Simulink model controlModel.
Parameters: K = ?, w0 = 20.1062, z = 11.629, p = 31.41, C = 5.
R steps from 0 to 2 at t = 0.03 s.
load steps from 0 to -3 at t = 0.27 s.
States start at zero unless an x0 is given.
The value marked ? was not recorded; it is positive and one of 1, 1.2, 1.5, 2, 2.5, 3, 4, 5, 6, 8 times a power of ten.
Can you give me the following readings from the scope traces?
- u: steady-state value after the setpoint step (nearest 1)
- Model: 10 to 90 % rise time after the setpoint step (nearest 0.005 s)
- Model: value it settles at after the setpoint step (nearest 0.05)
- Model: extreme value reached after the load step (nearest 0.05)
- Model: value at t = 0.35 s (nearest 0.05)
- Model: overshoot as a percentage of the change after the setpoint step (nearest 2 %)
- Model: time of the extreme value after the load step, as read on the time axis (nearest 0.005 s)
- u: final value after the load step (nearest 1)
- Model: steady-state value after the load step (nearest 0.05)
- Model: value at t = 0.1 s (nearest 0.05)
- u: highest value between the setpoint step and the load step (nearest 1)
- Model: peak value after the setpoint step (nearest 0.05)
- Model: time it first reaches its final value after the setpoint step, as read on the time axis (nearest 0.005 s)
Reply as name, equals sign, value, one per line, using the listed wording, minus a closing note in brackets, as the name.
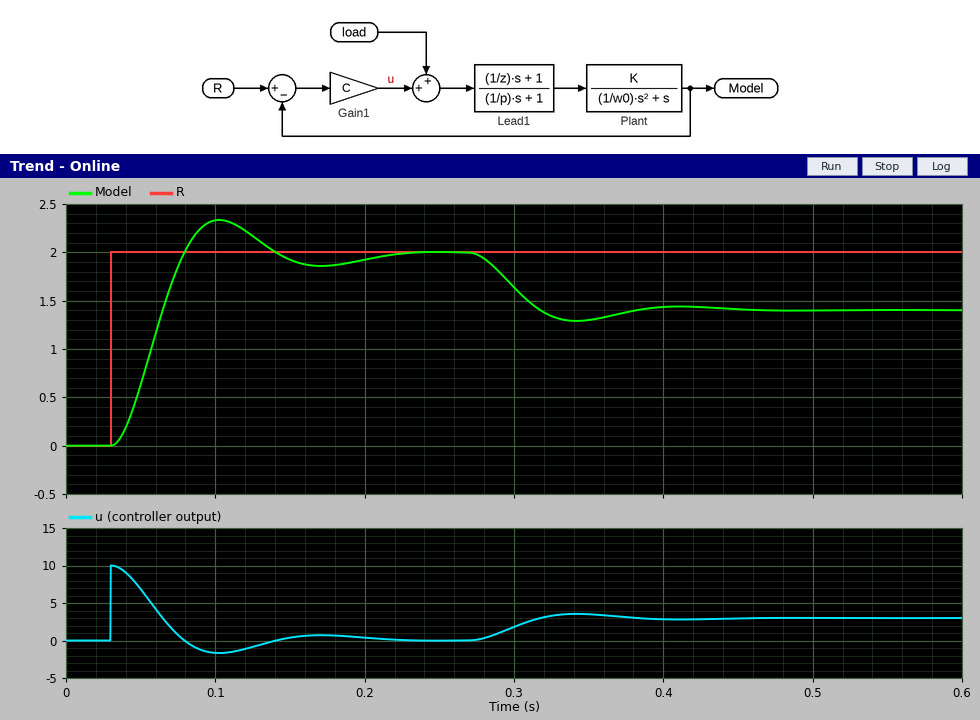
u: steady-state value after the setpoint step = 0
Model: 10 to 90 % rise time after the setpoint step = 0.035 s
Model: value it settles at after the setpoint step = 2.00
Model: extreme value reached after the load step = 1.30
Model: value at t = 0.35 s = 1.30
Model: overshoot as a percentage of the change after the setpoint step = 16 %
Model: time of the extreme value after the load step, as read on the time axis = 0.340 s
u: final value after the load step = 3
Model: steady-state value after the load step = 1.40
Model: value at t = 0.1 s = 2.35
u: highest value between the setpoint step and the load step = 10
Model: peak value after the setpoint step = 2.35
Model: time it first reaches its final value after the setpoint step, as read on the time axis = 0.080 s
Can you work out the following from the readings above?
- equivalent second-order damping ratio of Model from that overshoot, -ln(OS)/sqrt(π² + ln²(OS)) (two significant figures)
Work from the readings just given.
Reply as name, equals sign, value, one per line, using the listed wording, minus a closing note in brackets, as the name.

equivalent second-order damping ratio of Model from that overshoot, -ln(OS)/sqrt(π² + ln²(OS)) = 0.50
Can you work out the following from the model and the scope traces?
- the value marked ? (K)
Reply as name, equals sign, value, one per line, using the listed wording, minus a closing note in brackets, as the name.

the value marked ? = 8
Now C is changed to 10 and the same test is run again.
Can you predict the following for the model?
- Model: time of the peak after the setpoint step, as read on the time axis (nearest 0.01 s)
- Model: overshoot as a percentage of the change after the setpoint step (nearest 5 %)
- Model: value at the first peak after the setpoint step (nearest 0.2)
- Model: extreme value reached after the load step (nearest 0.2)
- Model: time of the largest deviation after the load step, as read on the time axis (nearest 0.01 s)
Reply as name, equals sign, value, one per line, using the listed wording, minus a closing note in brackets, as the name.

Model: time of the peak after the setpoint step, as read on the time axis = 0.08 s
Model: overshoot as a percentage of the change after the setpoint step = 35 %
Model: value at the first peak after the setpoint step = 2.6
Model: extreme value reached after the load step = 1.6
Model: time of the largest deviation after the load step, as read on the time axis = 0.32 s
